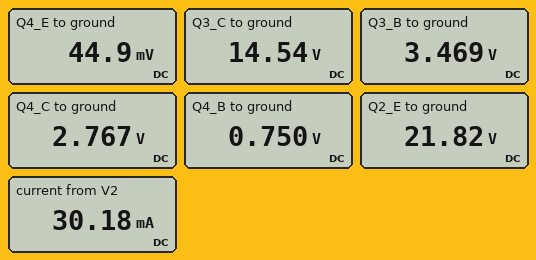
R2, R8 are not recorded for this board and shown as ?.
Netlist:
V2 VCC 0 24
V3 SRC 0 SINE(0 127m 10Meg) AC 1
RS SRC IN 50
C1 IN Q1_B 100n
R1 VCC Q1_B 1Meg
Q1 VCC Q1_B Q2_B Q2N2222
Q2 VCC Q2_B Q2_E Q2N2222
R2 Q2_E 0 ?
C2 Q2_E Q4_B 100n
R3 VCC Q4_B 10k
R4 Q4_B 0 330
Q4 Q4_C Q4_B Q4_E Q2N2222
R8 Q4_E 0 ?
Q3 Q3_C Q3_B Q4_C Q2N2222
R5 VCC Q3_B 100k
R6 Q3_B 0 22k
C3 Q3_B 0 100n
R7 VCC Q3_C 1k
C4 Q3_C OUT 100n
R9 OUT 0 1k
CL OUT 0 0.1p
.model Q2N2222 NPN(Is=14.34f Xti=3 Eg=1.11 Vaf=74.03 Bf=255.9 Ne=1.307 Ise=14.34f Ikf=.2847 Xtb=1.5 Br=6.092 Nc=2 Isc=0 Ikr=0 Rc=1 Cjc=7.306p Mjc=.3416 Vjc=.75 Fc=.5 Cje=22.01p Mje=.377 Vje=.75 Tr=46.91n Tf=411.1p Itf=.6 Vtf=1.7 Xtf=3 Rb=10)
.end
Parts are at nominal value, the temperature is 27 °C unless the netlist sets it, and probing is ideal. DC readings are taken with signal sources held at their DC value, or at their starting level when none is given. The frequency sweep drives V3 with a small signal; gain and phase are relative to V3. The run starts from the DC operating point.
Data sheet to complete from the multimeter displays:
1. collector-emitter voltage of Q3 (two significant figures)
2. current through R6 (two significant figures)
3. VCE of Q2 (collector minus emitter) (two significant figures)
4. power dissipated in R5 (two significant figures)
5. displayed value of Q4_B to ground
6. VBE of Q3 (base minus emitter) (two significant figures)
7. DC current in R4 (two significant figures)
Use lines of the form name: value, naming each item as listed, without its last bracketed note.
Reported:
collector-emitter voltage of Q3: 12 V
current through R6: 160 µA
VCE of Q2 (collector minus emitter): 2.2 V
power dissipated in R5: 4.2 mW
displayed value of Q4_B to ground: 0.750 V
VBE of Q3 (base minus emitter): 700 mV
DC current in R4: 2.3 mA
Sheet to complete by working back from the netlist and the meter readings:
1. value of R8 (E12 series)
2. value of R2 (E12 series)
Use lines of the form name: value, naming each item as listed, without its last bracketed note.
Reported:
value of R8: 4.7 Ω
value of R2: 1.2 kΩ
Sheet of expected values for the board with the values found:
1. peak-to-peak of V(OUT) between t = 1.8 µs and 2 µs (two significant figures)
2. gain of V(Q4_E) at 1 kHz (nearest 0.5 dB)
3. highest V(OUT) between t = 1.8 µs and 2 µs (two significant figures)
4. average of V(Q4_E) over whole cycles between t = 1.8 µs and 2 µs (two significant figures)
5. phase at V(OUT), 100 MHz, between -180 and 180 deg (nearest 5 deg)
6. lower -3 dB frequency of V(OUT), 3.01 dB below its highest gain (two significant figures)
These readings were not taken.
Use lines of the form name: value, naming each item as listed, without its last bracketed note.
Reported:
peak-to-peak of V(OUT) between t = 1.8 µs and 2 µs: 14 V
gain of V(Q4_E) at 1 kHz: -20.0 dB
highest V(OUT) between t = 1.8 µs and 2 µs: 4.5 V
average of V(Q4_E) over whole cycles between t = 1.8 µs and 2 µs: 58 mV
phase at V(OUT), 100 MHz, between -180 and 180 deg: 20 deg
lower -3 dB frequency of V(OUT), 3.01 dB below its highest gain: 6.1 kHz
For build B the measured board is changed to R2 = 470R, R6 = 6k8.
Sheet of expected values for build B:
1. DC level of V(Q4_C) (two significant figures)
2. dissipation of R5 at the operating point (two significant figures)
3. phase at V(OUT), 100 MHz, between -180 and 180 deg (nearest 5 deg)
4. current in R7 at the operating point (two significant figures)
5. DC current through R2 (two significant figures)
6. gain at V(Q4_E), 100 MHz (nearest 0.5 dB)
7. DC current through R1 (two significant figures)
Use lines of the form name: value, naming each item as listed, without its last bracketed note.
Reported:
DC level of V(Q4_C): 540 mV
dissipation of R5 at the operating point: 5.2 mW
phase at V(OUT), 100 MHz, between -180 and 180 deg: 10 deg
current in R7 at the operating point: 9.3 mA
DC current through R2: 44 mA
gain at V(Q4_E), 100 MHz: -9.0 dB
DC current through R1: 1.9 µA
